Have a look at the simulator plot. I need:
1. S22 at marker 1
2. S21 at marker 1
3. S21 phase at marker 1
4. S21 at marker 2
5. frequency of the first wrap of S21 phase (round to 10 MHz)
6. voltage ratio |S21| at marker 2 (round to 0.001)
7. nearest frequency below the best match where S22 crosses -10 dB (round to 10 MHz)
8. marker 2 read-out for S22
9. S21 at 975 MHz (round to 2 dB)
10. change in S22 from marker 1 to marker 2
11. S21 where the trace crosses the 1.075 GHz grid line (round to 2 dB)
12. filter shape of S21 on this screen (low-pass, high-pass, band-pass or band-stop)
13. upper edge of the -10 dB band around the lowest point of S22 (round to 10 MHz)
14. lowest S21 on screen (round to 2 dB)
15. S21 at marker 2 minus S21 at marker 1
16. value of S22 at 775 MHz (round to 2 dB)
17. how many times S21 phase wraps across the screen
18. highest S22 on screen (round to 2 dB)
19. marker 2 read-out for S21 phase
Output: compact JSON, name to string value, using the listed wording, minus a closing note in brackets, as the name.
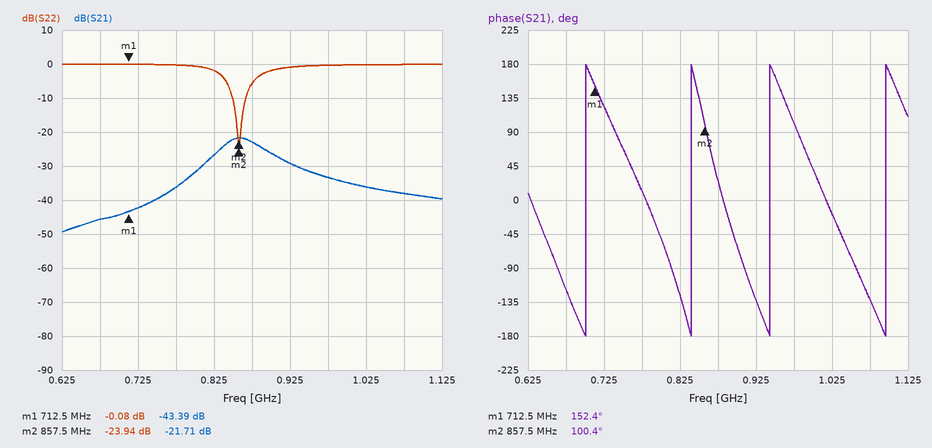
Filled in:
{"S22 at marker 1": "-0.08 dB", "S21 at marker 1": "-43.39 dB", "S21 phase at marker 1": "152.4°", "S21 at marker 2": "-21.71 dB", "frequency of the first wrap of S21 phase": "700 MHz", "voltage ratio |S21| at marker 2": "0.082", "nearest frequency below the best match where S22 crosses -10 dB": "850 MHz", "marker 2 read-out for S22": "-23.94 dB", "S21 at 975 MHz": "-34 dB", "change in S22 from marker 1 to marker 2": "-23.86 dB", "S21 where the trace crosses the 1.075 GHz grid line": "-38 dB", "filter shape of S21 on this screen": "band-pass", "upper edge of the -10 dB band around the lowest point of S22": "870 MHz", "lowest S21 on screen": "-50 dB", "S21 at marker 2 minus S21 at marker 1": "21.68 dB", "value of S22 at 775 MHz": "0 dB", "how many times S21 phase wraps across the screen": "4", "highest S22 on screen": "0 dB", "marker 2 read-out for S21 phase": "100.4°"}
